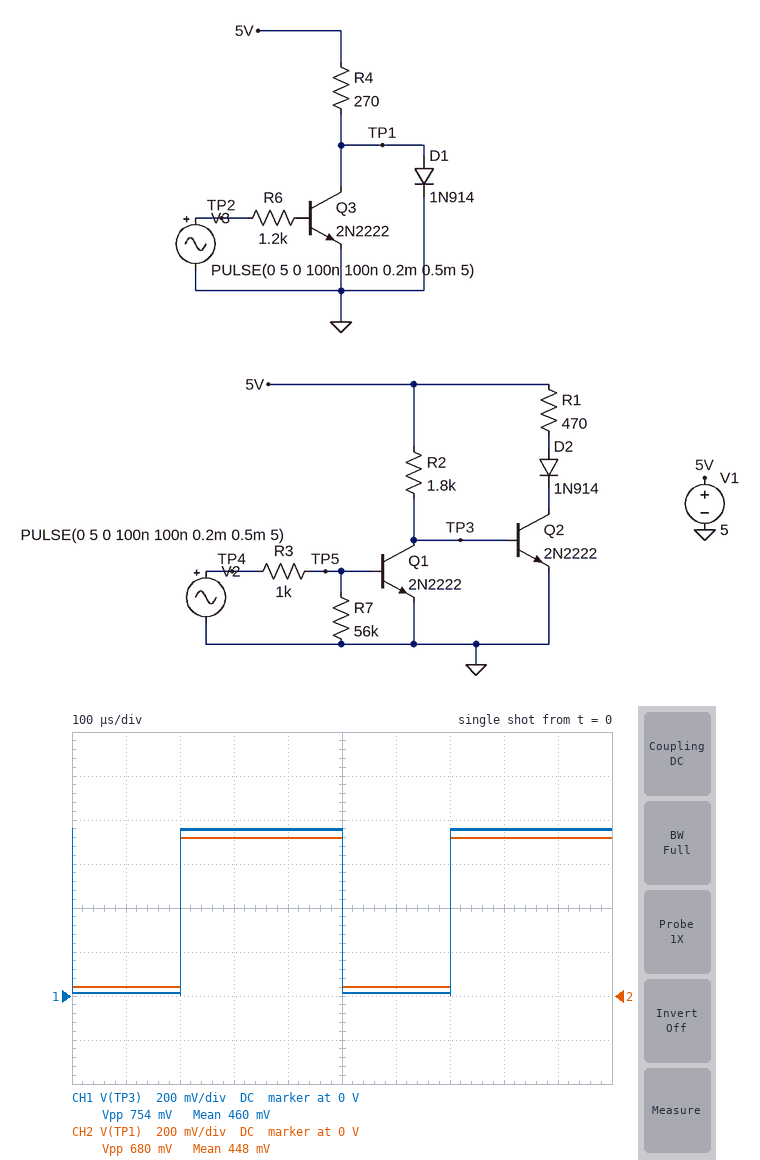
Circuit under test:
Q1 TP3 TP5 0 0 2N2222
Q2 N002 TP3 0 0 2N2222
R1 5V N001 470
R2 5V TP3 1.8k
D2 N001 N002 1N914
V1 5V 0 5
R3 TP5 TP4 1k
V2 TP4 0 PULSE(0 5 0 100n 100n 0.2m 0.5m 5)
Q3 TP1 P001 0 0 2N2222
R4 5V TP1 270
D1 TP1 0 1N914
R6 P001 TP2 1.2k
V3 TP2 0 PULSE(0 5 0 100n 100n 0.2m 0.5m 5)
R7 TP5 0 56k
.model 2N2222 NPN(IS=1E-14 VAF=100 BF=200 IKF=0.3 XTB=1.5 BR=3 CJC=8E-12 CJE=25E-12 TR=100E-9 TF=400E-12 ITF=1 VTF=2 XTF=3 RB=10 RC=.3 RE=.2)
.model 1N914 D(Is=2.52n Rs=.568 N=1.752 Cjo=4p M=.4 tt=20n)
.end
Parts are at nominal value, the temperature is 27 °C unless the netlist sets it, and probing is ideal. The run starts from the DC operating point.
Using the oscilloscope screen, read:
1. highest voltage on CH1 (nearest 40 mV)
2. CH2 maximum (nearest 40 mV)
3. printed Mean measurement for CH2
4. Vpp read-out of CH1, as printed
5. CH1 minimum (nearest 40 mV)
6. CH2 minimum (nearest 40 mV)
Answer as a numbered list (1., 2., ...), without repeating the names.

1. 760 mV
2. 720 mV
3. 448 mV
4. 754 mV
5. 0 V
6. 40 mV
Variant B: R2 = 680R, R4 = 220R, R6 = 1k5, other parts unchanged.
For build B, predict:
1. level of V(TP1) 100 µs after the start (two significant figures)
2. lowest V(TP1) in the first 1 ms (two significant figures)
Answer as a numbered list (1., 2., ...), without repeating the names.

1. 51 mV
2. 50 mV
